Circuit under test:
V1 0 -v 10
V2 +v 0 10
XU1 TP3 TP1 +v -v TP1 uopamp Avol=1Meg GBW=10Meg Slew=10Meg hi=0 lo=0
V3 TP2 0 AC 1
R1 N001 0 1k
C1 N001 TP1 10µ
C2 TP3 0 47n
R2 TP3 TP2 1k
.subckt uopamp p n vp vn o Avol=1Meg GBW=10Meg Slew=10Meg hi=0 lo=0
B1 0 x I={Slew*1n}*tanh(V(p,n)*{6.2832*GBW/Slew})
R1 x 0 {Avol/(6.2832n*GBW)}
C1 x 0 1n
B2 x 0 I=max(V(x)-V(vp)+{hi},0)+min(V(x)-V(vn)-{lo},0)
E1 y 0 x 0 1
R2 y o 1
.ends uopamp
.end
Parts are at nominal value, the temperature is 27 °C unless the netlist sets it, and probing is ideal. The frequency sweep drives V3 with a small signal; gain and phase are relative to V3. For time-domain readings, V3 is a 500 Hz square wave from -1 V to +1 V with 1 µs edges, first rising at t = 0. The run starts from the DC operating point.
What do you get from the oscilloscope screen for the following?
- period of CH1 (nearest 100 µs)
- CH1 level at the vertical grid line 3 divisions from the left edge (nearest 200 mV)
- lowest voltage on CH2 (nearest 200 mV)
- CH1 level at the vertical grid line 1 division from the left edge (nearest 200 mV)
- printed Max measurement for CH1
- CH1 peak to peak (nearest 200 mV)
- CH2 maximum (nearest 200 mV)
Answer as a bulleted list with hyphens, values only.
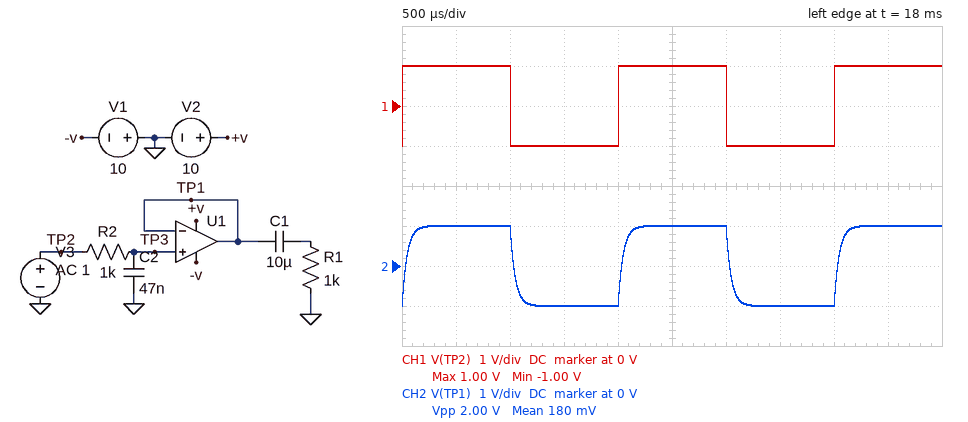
- 2.0 ms
- -1.0 V
- -1.0 V
- 1.0 V
- 1.00 V
- 2.0 V
- 1.0 V
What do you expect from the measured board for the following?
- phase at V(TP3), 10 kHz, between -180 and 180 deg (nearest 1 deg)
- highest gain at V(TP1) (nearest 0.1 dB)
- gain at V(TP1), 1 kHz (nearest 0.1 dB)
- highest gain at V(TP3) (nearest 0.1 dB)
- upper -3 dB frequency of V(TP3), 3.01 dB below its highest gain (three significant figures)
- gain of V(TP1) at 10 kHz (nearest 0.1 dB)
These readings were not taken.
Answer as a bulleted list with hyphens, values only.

- -71 deg
- 0 dB
- -0.4 dB
- 0 dB
- 3.39 kHz
- -9.9 dB
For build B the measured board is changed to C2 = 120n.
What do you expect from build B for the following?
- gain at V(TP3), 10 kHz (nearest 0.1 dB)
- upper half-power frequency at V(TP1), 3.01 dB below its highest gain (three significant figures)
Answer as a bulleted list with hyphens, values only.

- -17.6 dB
- 1.33 kHz
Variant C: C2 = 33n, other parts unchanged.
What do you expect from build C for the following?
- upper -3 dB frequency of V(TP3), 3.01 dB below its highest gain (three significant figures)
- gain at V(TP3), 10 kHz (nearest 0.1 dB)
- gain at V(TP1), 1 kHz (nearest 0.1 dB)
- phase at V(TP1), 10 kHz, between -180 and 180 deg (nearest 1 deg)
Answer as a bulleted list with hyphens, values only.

- 4.82 kHz
- -7.2 dB
- -0.2 dB
- -64 deg
